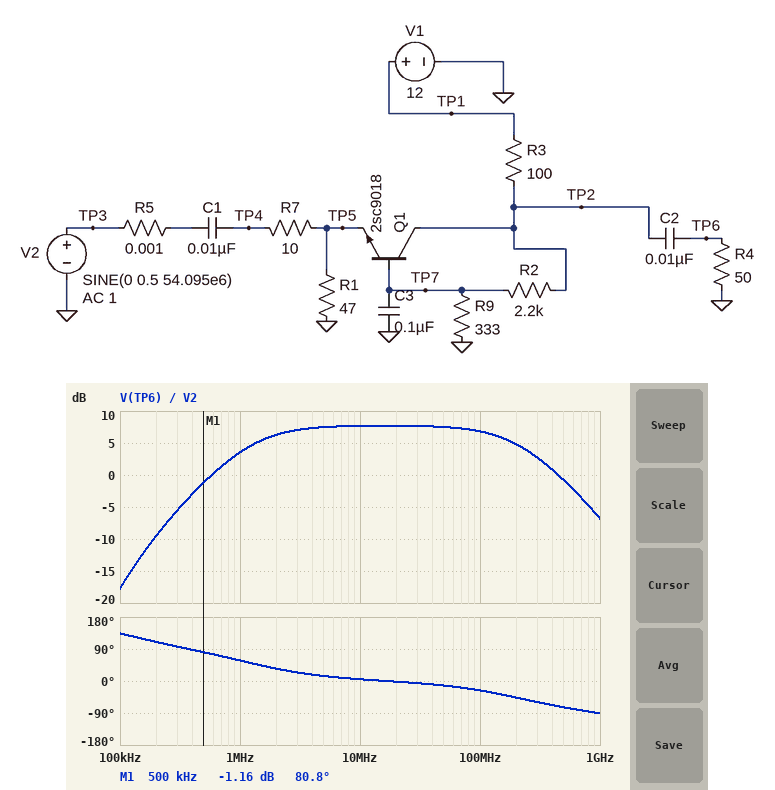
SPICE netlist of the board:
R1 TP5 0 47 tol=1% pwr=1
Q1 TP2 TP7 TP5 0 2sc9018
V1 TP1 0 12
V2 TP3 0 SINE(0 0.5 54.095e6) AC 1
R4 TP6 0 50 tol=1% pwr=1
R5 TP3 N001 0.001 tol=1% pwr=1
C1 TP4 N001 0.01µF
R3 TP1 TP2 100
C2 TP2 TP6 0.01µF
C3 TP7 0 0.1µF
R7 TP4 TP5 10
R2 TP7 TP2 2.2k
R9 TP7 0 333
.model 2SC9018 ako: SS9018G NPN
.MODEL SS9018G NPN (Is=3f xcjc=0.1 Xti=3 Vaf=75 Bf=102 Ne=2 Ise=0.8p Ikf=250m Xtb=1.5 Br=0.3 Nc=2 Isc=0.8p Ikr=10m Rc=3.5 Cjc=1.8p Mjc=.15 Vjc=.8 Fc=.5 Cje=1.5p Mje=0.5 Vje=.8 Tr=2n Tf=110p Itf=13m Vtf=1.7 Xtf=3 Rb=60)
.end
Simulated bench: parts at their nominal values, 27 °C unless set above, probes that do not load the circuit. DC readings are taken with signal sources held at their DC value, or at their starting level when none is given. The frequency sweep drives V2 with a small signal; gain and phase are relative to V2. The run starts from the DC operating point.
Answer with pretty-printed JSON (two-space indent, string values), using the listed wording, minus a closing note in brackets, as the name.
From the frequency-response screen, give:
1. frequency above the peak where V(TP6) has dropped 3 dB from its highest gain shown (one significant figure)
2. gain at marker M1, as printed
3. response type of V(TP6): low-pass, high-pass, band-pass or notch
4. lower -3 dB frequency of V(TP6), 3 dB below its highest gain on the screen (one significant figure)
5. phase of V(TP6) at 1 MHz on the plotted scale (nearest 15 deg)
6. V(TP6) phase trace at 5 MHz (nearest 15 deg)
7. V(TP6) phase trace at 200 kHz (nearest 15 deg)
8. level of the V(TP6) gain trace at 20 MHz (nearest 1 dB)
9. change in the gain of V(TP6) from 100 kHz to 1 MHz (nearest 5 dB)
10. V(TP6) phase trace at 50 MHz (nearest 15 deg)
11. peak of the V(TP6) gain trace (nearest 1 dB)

{
  "frequency above the peak where V(TP6) has dropped 3 dB from its highest gain shown": "200 MHz",
  "gain at marker M1, as printed": "-1.16 dB",
  "response type of V(TP6): low-pass, high-pass, band-pass or notch": "band-pass",
  "lower -3 dB frequency of V(TP6), 3 dB below its highest gain on the screen": "1 MHz",
  "phase of V(TP6) at 1 MHz on the plotted scale": "60 deg",
  "V(TP6) phase trace at 5 MHz": "15 deg",
  "V(TP6) phase trace at 200 kHz": "105 deg",
  "level of the V(TP6) gain trace at 20 MHz": "8 dB",
  "change in the gain of V(TP6) from 100 kHz to 1 MHz": "20 dB",
  "V(TP6) phase trace at 50 MHz": "-15 deg",
  "peak of the V(TP6) gain trace": "8 dB"
}
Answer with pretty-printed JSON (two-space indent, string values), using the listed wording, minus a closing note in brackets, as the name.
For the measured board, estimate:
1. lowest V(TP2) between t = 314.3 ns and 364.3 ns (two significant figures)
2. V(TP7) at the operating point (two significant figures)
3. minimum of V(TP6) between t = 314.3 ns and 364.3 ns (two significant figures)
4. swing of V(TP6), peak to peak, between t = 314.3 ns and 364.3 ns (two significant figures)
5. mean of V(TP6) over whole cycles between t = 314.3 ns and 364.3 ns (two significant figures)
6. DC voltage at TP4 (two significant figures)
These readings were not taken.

{
  "lowest V(TP2) between t = 314.3 ns and 364.3 ns": "9.3 V",
  "V(TP7) at the operating point": "1.3 V",
  "minimum of V(TP6) between t = 314.3 ns and 364.3 ns": "-1.0 V",
  "swing of V(TP6), peak to peak, between t = 314.3 ns and 364.3 ns": "1.4 V",
  "mean of V(TP6) over whole cycles between t = 314.3 ns and 364.3 ns": "-73 mV",
  "DC voltage at TP4": "580 mV"
}
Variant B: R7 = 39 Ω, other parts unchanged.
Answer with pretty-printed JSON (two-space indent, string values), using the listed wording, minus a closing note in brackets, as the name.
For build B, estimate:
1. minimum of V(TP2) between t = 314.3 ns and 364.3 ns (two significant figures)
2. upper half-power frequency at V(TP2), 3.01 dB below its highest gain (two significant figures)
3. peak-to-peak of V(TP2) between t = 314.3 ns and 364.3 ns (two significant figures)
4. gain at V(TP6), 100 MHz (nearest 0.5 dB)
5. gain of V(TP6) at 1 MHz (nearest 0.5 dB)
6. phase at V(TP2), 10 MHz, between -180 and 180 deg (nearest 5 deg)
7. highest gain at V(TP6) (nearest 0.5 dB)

{
  "minimum of V(TP2) between t = 314.3 ns and 364.3 ns": "10 V",
  "upper half-power frequency at V(TP2), 3.01 dB below its highest gain": "370 MHz",
  "peak-to-peak of V(TP2) between t = 314.3 ns and 364.3 ns": "710 mV",
  "gain at V(TP6), 100 MHz": "-3.0 dB",
  "gain of V(TP6) at 1 MHz": "-3.5 dB",
  "phase at V(TP2), 10 MHz, between -180 and 180 deg": "0 deg",
  "highest gain at V(TP6)": "-2.5 dB"
}
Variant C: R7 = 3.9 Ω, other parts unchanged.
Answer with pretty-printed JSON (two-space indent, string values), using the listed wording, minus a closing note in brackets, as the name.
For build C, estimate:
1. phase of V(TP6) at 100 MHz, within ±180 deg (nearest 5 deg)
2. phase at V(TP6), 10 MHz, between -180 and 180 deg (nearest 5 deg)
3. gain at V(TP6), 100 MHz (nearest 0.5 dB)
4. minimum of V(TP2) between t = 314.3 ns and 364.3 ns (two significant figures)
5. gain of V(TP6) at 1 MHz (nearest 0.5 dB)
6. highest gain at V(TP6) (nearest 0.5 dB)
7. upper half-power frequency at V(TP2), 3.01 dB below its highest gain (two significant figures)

{
  "phase of V(TP6) at 100 MHz, within ±180 deg": "-40 deg",
  "phase at V(TP6), 10 MHz, between -180 and 180 deg": "10 deg",
  "gain at V(TP6), 100 MHz": "11.5 dB",
  "minimum of V(TP2) between t = 314.3 ns and 364.3 ns": "8.8 V",
  "gain of V(TP6) at 1 MHz": "5.0 dB",
  "highest gain at V(TP6)": "13.5 dB",
  "upper half-power frequency at V(TP2), 3.01 dB below its highest gain": "130 MHz"
}
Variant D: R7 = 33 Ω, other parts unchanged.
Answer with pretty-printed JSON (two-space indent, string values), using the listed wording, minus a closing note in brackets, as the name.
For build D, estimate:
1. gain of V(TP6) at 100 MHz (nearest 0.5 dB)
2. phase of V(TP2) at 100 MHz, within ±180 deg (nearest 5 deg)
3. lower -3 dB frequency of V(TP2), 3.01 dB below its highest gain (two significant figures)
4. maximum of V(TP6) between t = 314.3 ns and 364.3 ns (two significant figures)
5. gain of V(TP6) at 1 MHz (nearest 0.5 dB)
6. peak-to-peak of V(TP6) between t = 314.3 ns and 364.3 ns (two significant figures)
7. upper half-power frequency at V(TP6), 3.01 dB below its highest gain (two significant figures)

{
  "gain of V(TP6) at 100 MHz": "-1.5 dB",
  "phase of V(TP2) at 100 MHz, within ±180 deg": "-15 deg",
  "lower -3 dB frequency of V(TP2), 3.01 dB below its highest gain": "230 kHz",
  "maximum of V(TP6) between t = 314.3 ns and 364.3 ns": "370 mV",
  "gain of V(TP6) at 1 MHz": "-2.0 dB",
  "peak-to-peak of V(TP6) between t = 314.3 ns and 364.3 ns": "800 mV",
  "upper half-power frequency at V(TP6), 3.01 dB below its highest gain": "350 MHz"
}
